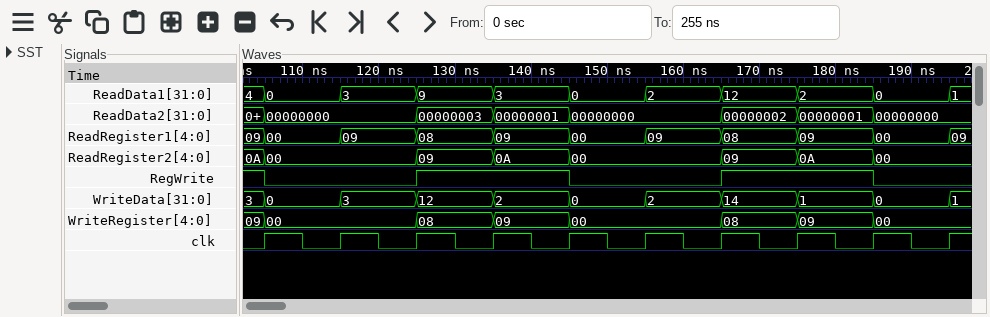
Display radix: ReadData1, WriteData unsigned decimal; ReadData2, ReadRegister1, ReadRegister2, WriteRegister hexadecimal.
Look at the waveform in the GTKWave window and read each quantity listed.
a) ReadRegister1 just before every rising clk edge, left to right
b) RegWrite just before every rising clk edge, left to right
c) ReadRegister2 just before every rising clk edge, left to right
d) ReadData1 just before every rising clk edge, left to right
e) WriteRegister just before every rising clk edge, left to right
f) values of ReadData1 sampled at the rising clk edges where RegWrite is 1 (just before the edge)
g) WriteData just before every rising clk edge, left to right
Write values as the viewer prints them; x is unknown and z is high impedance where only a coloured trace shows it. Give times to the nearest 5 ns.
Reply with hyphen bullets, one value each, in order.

- 09, 00, 09, 08, 09, 00, 09, 08, 09, 00
- 1 0 0 1 1 0 0 1 1 0
- 0A, 00, 00, 09, 0A, 00, 00, 09, 0A, 00
- 4, 0, 3, 9, 3, 0, 2, 12, 2, 0
- 09, 00, 00, 08, 09, 00, 00, 08, 09, 00
- 4, 9, 3, 12, 2
- 3, 0, 3, 12, 2, 0, 2, 14, 1, 0
